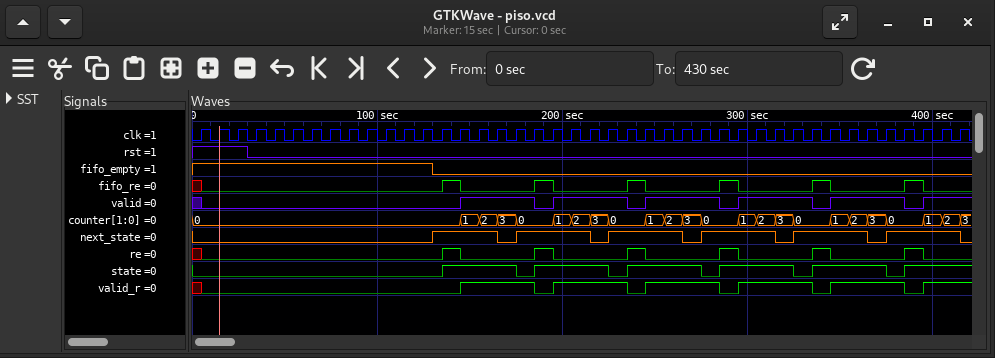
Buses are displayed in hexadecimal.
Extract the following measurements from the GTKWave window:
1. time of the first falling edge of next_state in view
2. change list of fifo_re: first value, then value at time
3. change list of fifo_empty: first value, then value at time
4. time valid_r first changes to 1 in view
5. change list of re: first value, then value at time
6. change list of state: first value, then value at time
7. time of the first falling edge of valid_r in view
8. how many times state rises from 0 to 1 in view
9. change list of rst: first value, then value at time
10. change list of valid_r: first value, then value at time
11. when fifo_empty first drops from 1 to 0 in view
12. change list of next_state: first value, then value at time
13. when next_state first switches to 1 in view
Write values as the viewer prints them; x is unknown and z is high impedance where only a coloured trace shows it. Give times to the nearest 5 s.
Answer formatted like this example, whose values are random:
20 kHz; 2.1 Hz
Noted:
165 s; x, 0 at 5 s, 1 at 135 s, 0 at 145 s, 1 at 185 s, 0 at 195 s, 1 at 235 s, 0 at 245 s, 1 at 285 s, 0 at 295 s, 1 at 335 s, 0 at 345 s, 1 at 385 s, 0 at 395 s; 1, 0 at 130 s; 145 s; x, 0 at 5 s, 1 at 135 s, 0 at 145 s, 1 at 185 s, 0 at 195 s, 1 at 235 s, 0 at 245 s, 1 at 285 s, 0 at 295 s, 1 at 335 s, 0 at 345 s, 1 at 385 s, 0 at 395 s; 0, 1 at 135 s, 0 at 175 s, 1 at 185 s, 0 at 225 s, 1 at 235 s, 0 at 275 s, 1 at 285 s, 0 at 325 s, 1 at 335 s, 0 at 375 s, 1 at 385 s; 185 s; 6; 1, 0 at 30 s; x, 0 at 5 s, 1 at 145 s, 0 at 185 s, 1 at 195 s, 0 at 235 s, 1 at 245 s, 0 at 285 s, 1 at 295 s, 0 at 335 s, 1 at 345 s, 0 at 385 s, 1 at 395 s; 130 s; 0, 1 at 130 s, 0 at 165 s, 1 at 175 s, 0 at 215 s, 1 at 225 s, 0 at 265 s, 1 at 275 s, 0 at 315 s, 1 at 325 s, 0 at 365 s, 1 at 375 s, 0 at 415 s; 130 s
